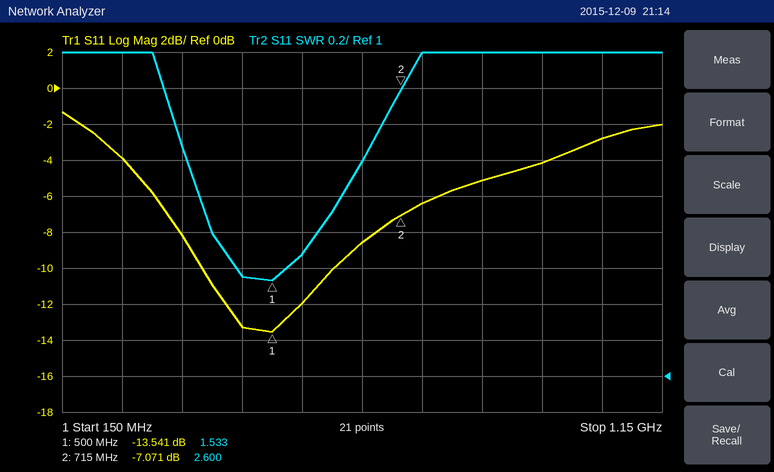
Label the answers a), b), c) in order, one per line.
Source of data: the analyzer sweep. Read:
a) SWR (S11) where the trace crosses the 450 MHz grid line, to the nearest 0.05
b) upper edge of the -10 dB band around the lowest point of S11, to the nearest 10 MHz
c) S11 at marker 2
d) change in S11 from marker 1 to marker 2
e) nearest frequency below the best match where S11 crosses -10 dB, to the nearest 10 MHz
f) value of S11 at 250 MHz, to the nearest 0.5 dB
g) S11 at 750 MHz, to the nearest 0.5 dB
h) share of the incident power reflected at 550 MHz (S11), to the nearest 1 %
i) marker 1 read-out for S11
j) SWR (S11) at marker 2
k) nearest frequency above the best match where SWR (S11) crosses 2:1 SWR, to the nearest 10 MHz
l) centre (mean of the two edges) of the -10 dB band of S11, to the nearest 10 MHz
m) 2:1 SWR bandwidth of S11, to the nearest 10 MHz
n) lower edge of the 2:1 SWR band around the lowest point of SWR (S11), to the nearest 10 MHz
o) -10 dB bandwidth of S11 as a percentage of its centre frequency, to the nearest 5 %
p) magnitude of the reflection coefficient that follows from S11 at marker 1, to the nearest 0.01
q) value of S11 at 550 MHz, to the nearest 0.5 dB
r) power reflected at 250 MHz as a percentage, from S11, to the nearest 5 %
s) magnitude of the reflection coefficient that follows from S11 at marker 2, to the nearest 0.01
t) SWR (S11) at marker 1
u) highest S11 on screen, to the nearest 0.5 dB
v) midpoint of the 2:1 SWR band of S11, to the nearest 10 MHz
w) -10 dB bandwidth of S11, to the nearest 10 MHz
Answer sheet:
a) 1.55
b) 600 MHz
c) -7.071 dB
d) 6.470 dB
e) 380 MHz
f) -4.0 dB
g) -6.5 dB
h) 6 %
i) -13.541 dB
j) 2.600
k) 620 MHz
l) 490 MHz
m) 240 MHz
n) 380 MHz
o) 45 %
p) 0.21
q) -12.0 dB
r) 40 %
s) 0.44
t) 1.533
u) -1.5 dB
v) 500 MHz
w) 220 MHz
